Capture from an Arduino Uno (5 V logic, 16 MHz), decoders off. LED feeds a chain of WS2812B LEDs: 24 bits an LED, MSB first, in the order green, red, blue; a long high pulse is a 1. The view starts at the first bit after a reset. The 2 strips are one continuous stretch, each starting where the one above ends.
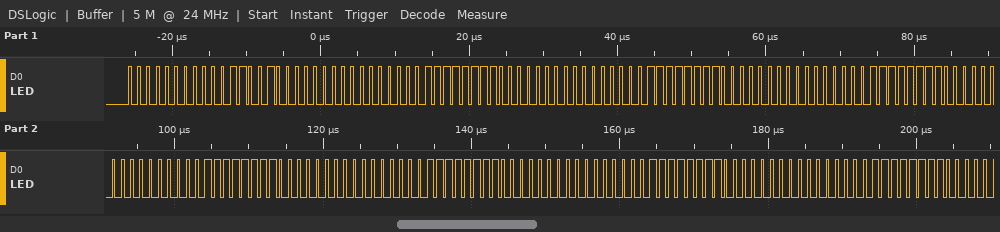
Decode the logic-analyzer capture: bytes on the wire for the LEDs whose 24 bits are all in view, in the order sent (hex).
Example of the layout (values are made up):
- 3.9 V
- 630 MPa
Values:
- 00 19 00 00 FF 00 00 FF 00 00 FF 00 00 FF 00 00 FF 00 00 FF 00
